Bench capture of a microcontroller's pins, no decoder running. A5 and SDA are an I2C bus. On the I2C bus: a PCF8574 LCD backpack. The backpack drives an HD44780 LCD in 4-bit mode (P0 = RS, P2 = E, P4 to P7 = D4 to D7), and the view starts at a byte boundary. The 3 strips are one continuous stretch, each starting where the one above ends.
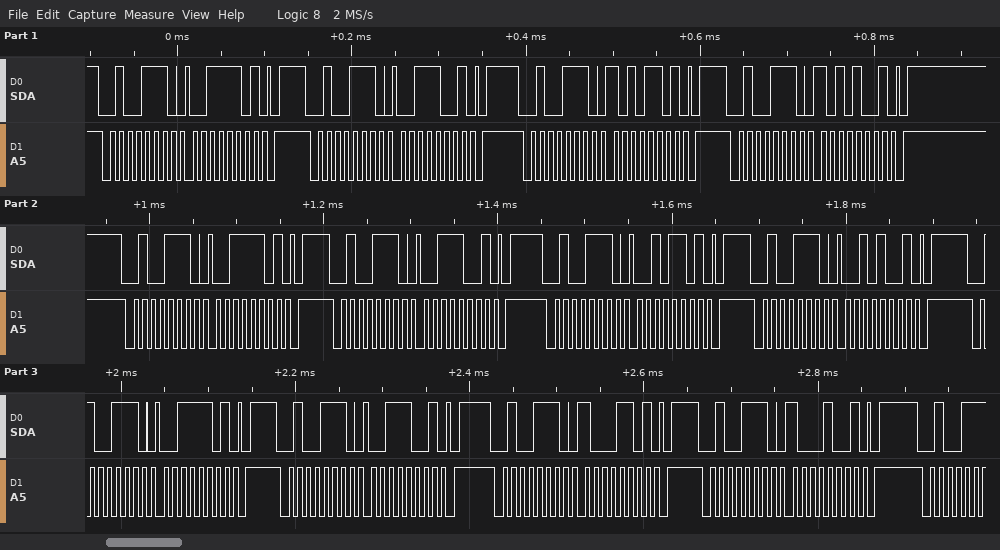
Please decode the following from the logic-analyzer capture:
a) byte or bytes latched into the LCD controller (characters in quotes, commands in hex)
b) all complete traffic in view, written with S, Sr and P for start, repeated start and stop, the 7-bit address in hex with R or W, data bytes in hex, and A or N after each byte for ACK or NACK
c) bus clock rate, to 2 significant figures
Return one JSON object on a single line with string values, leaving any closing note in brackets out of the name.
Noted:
{"byte or bytes latched into the LCD controller": "':' '2' '8'", "all complete traffic in view, written with S, Sr and P for start, repeated start and stop, the 7-bit address in hex with R or W, data bytes in hex, and A or N after each byte for ACK or NACK": "S 27W A 3D A P S 27W A 39 A P S 27W A AD A P S 27W A A9 A P S 27W A 3D A P S 27W A 39 A P S 27W A 2D A P S 27W A 29 A P S 27W A 3D A P S 27W A 39 A P S 27W A 8D A P S 27W A 89 A P", "bus clock rate, to 2 significant figures": "100 kHz"}
